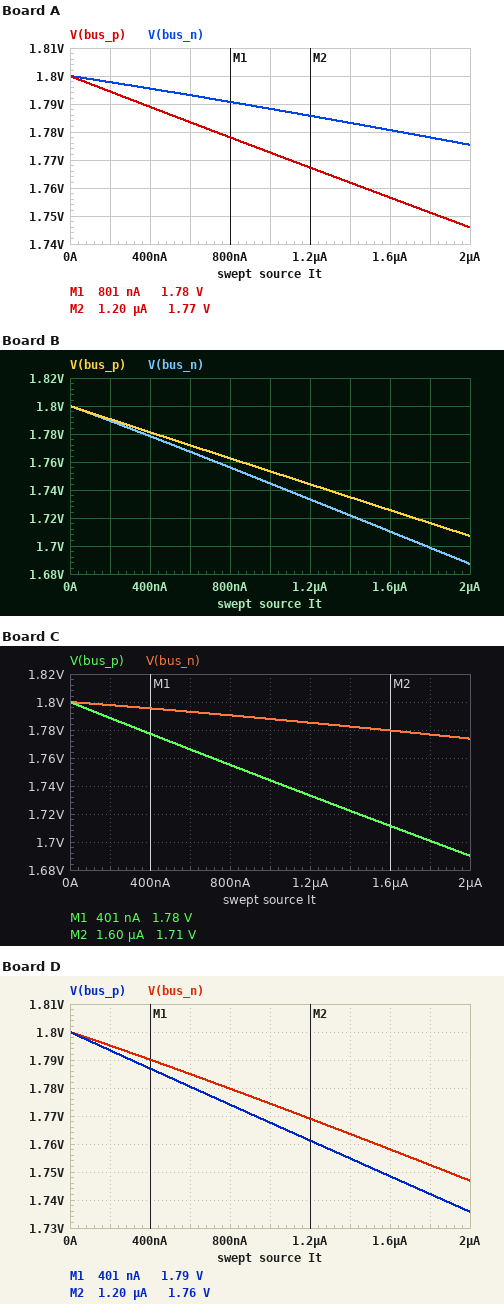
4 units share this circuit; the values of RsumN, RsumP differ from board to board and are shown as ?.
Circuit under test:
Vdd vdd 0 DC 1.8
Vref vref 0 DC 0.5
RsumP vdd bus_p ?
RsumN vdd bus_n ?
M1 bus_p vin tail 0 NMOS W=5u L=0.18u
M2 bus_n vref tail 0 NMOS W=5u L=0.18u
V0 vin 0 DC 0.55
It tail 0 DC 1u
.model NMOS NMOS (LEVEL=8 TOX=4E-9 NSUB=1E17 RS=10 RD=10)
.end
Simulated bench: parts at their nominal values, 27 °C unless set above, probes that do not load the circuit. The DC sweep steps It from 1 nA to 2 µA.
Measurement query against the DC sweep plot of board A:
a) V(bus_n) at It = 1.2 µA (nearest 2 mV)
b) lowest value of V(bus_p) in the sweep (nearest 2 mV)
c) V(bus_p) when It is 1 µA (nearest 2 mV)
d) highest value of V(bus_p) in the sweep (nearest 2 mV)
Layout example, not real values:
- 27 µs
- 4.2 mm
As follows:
- 1.786 V
- 1.746 V
- 1.772 V
- 1.800 V
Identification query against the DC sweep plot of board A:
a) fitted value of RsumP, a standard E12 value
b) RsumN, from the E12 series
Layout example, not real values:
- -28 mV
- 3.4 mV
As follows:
- 33 kΩ
- 68 kΩ
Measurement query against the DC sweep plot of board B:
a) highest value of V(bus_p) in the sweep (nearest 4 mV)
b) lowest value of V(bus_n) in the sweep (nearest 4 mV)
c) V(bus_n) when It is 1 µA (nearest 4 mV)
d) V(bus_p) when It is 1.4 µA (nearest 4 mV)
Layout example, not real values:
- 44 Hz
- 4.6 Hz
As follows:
- 1.800 V
- 1.688 V
- 1.744 V
- 1.736 V
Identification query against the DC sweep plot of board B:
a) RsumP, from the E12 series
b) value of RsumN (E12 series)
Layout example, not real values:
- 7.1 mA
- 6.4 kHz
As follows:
- 56 kΩ
- 330 kΩ
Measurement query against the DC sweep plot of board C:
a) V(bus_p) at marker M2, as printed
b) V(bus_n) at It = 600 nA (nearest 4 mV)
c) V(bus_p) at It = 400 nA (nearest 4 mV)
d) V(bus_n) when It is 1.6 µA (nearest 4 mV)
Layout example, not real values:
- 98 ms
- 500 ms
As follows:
- 1.71 V
- 1.792 V
- 1.776 V
- 1.780 V
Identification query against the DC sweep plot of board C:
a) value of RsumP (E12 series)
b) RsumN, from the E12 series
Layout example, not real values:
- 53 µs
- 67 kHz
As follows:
- 68 kΩ
- 68 kΩ
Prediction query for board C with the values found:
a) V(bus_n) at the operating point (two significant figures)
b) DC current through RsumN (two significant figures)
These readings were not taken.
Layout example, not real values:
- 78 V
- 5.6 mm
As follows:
- 1.8 V
- 180 nA
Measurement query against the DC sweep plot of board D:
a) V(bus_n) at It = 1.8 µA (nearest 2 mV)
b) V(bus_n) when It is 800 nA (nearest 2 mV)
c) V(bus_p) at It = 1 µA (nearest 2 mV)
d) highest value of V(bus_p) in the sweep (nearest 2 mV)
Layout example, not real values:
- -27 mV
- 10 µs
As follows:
- 1.752 V
- 1.780 V
- 1.768 V
- 1.800 V
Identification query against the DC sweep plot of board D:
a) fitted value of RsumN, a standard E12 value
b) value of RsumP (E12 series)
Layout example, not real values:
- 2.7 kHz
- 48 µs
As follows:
- 150 kΩ
- 39 kΩ
